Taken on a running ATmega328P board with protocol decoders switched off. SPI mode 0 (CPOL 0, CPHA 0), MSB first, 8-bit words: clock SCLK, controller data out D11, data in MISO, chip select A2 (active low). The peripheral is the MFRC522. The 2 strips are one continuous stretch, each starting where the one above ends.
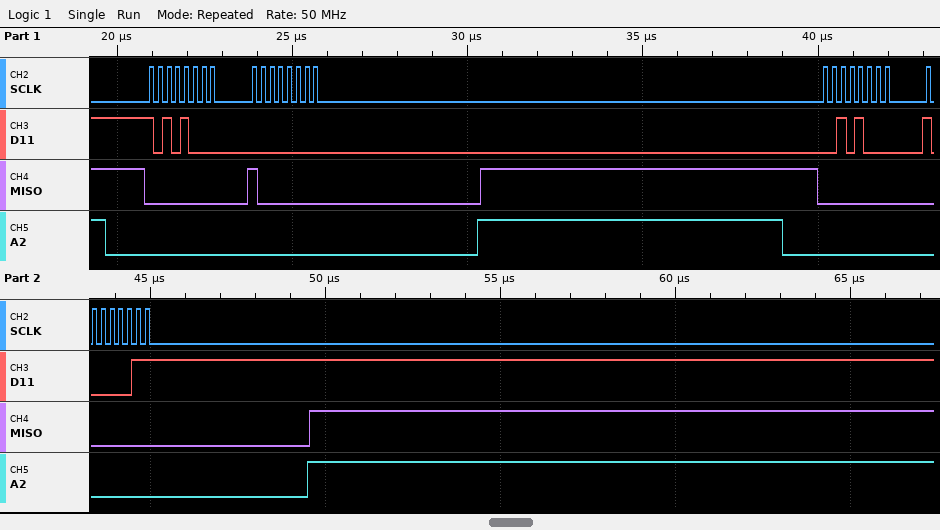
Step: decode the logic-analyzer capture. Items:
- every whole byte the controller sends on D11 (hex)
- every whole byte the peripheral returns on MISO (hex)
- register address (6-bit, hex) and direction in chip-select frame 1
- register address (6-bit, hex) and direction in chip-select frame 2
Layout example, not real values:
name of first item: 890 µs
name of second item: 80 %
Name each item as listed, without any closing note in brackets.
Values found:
every whole byte the controller sends on D11: 0xA8 0x00 0x28 0x83
every whole byte the peripheral returns on MISO: 0x00 0x80 0x00 0x00
register address (6-bit, hex) and direction in chip-select frame 1: 0x14 read
register address (6-bit, hex) and direction in chip-select frame 2: 0x14 write
